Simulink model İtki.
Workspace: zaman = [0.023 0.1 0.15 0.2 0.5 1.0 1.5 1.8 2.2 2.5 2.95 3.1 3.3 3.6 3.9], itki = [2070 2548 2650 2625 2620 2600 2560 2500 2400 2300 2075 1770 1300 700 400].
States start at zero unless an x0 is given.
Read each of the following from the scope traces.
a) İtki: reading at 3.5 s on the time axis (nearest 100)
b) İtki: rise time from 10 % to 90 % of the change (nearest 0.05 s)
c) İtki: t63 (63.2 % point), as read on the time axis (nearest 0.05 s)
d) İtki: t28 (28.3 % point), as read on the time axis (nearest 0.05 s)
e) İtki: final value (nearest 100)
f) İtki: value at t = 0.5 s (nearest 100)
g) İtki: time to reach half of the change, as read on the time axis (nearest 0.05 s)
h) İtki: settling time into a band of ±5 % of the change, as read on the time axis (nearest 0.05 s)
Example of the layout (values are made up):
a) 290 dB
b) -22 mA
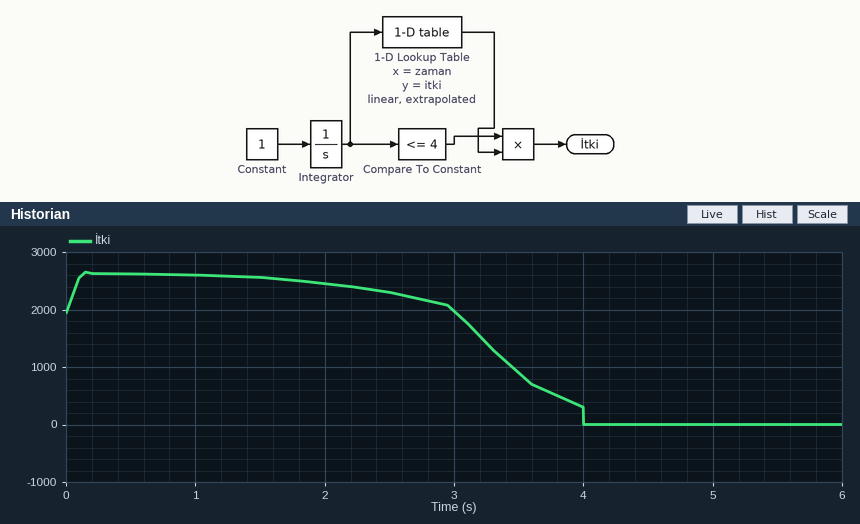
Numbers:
a) 900
b) 0.90 s
c) 3.60 s
d) 3.25 s
e) 0
f) 2600
g) 3.45 s
h) 4.00 s
